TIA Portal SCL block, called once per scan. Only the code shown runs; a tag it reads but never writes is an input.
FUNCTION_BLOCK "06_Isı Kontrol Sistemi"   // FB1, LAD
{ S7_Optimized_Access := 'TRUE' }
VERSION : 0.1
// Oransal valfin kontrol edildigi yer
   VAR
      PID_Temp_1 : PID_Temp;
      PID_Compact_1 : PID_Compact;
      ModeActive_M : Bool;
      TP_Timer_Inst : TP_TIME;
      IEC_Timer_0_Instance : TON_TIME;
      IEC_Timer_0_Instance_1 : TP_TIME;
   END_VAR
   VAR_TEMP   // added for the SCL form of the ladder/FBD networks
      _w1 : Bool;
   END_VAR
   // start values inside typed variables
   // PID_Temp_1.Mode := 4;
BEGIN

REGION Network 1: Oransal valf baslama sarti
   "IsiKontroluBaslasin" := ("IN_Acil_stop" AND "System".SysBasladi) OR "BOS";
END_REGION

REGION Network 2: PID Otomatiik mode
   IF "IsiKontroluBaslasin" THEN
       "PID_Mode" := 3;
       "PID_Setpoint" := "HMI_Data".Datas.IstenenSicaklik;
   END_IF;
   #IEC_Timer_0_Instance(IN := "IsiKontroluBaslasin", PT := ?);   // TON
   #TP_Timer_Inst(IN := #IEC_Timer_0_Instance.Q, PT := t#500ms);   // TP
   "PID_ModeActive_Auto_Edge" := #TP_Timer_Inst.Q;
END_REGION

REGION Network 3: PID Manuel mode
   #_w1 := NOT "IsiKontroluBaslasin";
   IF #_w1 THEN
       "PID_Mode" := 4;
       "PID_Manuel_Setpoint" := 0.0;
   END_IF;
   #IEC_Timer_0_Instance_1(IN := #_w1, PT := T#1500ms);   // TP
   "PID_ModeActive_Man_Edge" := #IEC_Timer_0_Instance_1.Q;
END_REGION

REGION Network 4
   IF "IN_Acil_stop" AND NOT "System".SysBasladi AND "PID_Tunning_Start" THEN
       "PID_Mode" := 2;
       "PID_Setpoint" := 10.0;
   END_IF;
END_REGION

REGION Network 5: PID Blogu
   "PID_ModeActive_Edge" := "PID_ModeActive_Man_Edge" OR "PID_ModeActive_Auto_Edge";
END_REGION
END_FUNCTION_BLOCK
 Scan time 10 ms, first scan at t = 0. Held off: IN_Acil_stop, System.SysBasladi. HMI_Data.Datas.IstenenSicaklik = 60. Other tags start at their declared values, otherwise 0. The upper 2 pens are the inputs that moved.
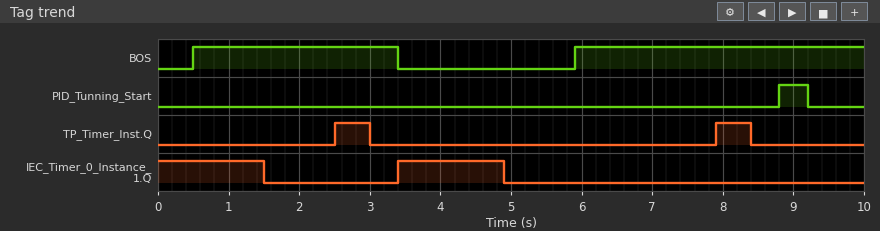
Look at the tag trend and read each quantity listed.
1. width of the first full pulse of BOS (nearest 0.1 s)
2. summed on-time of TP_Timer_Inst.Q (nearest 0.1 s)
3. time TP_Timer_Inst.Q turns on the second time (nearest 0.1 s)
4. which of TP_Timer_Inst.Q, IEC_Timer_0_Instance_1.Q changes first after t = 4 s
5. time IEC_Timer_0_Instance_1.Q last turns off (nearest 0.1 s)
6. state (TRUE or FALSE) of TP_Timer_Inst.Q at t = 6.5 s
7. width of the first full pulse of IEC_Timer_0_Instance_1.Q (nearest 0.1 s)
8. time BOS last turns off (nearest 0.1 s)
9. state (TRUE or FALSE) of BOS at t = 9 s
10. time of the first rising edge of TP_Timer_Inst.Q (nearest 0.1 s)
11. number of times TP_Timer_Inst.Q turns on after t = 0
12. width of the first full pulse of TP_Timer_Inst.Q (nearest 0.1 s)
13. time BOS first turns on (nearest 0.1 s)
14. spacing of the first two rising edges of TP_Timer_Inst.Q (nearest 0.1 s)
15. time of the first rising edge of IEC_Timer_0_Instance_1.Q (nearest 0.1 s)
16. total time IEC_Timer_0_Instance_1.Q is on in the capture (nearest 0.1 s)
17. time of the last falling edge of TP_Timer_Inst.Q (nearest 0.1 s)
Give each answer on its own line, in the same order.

2.9 s
1.0 s
7.9 s
IEC_Timer_0_Instance_1.Q
4.9 s
FALSE
1.5 s
3.4 s
TRUE
2.5 s
2
0.5 s
0.5 s
5.4 s
3.4 s
3.0 s
8.4 s
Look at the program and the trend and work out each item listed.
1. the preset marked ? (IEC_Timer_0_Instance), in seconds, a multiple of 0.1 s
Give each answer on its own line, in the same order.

2.0 s
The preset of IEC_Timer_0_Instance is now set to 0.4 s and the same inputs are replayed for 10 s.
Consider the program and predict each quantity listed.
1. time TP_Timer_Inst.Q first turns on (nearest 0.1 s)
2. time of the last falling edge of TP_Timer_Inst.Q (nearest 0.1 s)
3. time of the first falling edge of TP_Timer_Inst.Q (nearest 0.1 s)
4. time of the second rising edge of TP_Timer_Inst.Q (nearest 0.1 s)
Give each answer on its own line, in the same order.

0.9 s
6.8 s
1.4 s
6.3 s
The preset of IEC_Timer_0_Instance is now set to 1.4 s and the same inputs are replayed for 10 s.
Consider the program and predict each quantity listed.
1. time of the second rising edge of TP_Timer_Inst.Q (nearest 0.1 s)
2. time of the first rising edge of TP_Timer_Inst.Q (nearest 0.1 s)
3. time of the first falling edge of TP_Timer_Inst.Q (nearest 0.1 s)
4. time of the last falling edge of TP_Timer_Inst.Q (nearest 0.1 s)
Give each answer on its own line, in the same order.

7.3 s
1.9 s
2.4 s
7.8 s
